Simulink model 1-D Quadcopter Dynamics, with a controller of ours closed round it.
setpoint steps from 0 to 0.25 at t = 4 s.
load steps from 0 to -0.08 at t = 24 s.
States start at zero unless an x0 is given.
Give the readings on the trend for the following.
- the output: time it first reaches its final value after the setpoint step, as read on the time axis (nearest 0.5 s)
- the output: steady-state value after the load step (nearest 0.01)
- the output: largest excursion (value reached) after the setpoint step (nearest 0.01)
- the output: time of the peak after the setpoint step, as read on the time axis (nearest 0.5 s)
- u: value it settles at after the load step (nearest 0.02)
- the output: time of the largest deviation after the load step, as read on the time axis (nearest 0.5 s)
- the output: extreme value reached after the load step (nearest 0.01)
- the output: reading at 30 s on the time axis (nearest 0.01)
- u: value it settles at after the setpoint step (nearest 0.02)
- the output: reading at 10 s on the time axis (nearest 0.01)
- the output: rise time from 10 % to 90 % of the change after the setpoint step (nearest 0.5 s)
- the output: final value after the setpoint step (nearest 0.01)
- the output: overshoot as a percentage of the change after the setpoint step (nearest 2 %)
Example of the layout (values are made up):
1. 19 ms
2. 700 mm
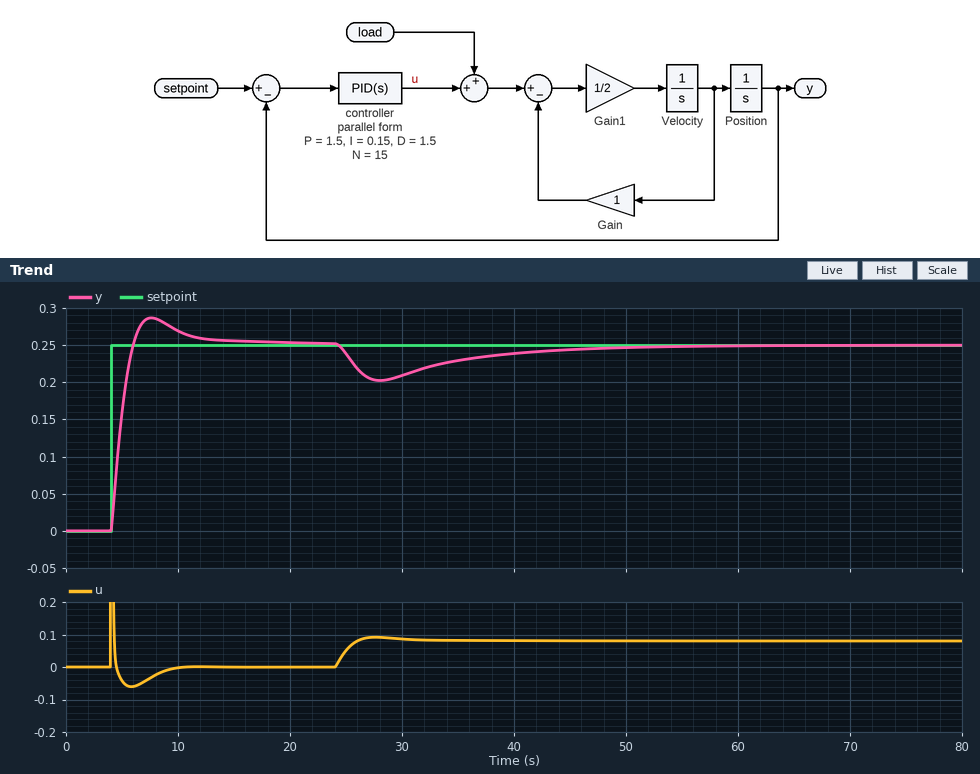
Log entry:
1. 6.0 s
2. 0.25
3. 0.29
4. 7.5 s
5. 0.08
6. 28.0 s
7. 0.20
8. 0.21
9. 0.00
10. 0.27
11. 1.5 s
12. 0.25
13. 14 %
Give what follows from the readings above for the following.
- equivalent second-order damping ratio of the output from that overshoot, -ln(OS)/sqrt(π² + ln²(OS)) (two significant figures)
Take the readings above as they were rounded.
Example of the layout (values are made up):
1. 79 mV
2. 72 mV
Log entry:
1. 0.53
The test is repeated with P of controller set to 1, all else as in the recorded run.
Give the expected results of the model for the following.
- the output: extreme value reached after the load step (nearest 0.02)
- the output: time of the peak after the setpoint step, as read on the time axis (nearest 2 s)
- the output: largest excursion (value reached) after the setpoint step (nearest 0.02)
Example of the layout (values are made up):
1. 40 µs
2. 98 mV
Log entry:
1. 0.18
2. 10 s
3. 0.28
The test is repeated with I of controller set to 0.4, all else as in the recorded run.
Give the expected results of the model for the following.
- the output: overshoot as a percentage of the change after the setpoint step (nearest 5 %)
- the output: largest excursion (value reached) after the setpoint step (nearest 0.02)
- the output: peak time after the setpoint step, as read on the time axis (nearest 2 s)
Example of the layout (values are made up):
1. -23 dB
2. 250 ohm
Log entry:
1. 25 %
2. 0.32
3. 8 s
